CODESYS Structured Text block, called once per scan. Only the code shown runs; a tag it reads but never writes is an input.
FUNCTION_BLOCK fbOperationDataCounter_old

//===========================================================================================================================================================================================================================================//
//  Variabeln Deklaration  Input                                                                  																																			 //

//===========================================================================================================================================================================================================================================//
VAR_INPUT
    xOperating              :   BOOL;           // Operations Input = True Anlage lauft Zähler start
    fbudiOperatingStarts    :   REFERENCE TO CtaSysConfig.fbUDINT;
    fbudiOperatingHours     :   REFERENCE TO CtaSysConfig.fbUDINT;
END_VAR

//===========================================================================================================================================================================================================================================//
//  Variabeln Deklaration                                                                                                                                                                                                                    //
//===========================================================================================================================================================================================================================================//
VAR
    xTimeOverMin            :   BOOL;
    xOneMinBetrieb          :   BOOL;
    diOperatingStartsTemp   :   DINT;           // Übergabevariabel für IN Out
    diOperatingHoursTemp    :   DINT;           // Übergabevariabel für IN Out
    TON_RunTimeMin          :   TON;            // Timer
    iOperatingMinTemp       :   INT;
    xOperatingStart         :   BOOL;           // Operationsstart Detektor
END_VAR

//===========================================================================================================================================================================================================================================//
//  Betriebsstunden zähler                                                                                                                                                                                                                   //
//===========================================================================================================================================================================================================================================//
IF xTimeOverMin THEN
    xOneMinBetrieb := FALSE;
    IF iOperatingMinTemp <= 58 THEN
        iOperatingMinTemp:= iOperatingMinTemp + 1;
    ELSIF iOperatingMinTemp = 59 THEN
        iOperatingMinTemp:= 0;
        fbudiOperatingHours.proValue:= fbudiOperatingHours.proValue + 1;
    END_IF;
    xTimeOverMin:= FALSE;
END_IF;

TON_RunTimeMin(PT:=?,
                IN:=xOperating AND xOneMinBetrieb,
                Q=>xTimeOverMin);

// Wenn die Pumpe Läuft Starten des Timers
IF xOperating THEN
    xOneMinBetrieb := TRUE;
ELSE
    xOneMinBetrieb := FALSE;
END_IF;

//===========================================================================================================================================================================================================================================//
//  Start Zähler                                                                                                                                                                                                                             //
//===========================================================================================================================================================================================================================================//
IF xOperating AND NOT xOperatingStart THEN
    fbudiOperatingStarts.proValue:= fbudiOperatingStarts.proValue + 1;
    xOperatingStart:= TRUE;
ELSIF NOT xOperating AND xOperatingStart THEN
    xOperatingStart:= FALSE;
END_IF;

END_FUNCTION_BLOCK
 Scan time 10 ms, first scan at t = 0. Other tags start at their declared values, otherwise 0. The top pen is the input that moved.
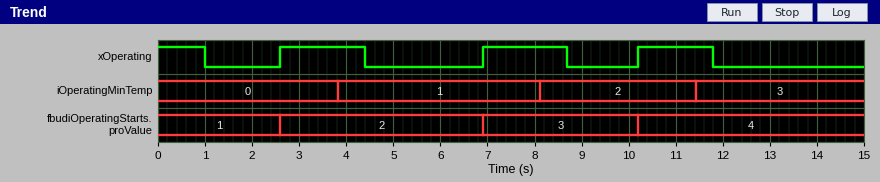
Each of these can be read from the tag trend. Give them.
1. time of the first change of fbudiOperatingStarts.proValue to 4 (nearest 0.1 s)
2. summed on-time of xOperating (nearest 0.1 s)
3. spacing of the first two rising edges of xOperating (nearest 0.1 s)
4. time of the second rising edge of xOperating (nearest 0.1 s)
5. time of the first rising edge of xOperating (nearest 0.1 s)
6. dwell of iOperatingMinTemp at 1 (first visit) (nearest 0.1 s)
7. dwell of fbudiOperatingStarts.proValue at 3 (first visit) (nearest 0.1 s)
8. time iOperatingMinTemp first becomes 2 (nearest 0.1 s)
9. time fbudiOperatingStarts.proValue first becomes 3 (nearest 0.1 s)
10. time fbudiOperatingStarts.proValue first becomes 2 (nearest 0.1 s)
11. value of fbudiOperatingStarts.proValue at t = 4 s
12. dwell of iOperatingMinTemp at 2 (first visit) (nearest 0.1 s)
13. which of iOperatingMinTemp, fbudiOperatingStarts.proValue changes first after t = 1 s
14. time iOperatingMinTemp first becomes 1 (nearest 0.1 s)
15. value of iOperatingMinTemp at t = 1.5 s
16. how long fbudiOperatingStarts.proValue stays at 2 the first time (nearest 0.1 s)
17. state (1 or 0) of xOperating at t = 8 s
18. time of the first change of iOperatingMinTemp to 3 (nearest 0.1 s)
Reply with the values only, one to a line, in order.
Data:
10.2 s
6.2 s
4.3 s
6.9 s
2.6 s
4.3 s
3.3 s
8.1 s
6.9 s
2.6 s
2
3.3 s
fbudiOperatingStarts.proValue
3.8 s
0
4.3 s
1
11.4 s
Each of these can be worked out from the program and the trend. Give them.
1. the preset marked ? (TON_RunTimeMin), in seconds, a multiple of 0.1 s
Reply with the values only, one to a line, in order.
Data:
1.2 s
